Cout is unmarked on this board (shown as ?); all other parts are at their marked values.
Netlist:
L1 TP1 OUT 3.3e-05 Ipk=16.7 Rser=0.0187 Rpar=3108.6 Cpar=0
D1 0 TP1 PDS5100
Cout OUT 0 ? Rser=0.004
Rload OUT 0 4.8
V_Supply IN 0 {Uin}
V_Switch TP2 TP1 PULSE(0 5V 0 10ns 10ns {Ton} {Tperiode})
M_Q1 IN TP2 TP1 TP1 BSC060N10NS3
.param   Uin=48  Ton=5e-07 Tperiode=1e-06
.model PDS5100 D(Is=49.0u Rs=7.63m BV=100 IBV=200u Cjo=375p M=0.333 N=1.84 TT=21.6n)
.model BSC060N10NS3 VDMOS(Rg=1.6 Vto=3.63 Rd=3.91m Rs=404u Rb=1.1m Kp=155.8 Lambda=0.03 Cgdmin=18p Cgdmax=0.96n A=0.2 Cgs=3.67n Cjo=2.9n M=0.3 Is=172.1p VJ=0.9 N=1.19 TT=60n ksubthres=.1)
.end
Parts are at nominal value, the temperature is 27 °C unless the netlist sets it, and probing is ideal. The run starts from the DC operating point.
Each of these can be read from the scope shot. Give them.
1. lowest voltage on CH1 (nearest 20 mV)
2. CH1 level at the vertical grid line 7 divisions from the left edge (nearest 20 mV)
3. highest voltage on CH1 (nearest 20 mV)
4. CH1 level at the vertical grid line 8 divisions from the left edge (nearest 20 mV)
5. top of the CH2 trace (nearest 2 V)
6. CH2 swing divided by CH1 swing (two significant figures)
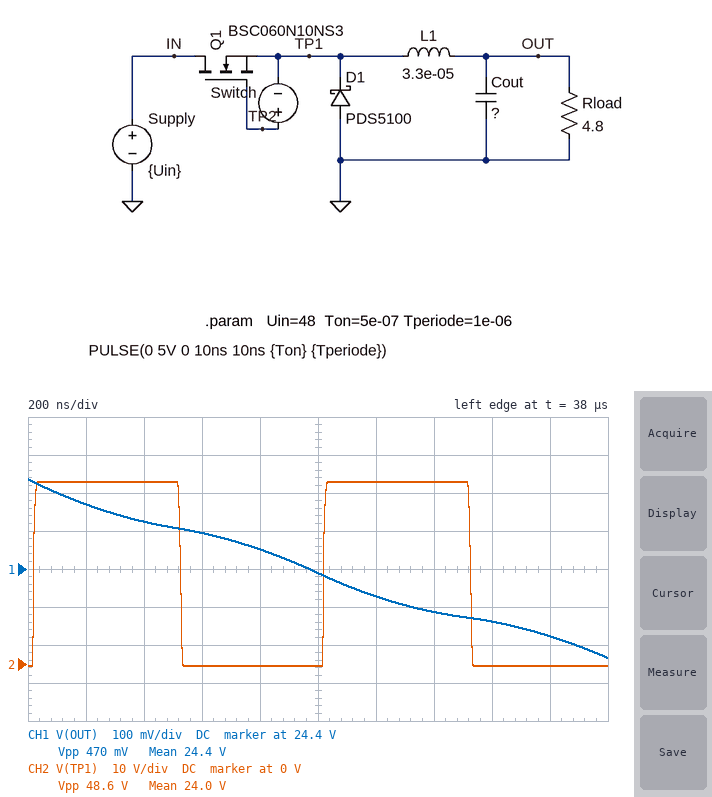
24.16 V
24.28 V
24.64 V
24.26 V
48 V
100
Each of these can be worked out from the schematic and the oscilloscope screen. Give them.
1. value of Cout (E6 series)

1.5 µF
